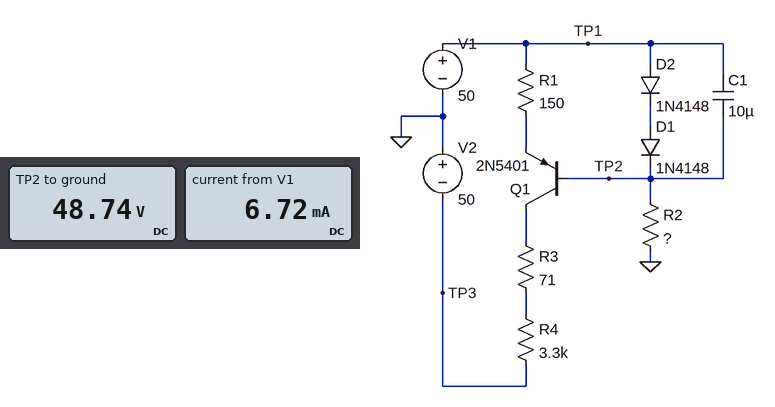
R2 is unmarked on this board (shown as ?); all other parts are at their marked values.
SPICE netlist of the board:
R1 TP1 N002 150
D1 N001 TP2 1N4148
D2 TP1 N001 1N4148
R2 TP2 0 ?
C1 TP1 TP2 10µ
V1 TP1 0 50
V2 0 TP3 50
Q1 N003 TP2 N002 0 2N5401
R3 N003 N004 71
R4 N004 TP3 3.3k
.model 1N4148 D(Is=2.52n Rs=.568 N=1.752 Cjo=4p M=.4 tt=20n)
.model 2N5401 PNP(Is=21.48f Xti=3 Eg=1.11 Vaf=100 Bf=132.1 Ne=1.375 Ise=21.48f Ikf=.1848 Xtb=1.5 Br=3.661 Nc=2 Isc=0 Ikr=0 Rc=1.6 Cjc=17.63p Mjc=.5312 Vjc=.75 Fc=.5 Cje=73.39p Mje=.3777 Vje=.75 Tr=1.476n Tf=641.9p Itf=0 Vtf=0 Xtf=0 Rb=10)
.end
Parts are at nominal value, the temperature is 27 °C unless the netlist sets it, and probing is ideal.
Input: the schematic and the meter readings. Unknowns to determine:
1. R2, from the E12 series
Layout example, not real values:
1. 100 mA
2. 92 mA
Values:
1. 18 kΩ
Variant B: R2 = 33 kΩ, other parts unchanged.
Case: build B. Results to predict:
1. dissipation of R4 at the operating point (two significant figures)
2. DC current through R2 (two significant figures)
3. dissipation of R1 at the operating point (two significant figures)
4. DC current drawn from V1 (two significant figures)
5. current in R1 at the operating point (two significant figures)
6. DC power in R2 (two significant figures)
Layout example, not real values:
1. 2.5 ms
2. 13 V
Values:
1. 44 mW
2. 1.5 mA
3. 2.0 mW
4. 5.1 mA
5. 3.7 mA
6. 72 mW
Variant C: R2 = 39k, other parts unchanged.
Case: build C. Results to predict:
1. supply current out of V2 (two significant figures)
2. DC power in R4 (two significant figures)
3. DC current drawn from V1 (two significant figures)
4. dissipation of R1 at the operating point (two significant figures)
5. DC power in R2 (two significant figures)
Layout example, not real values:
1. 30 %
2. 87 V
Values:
1. 3.6 mA
2. 42 mW
3. 4.8 mA
4. 1.9 mW
5. 61 mW
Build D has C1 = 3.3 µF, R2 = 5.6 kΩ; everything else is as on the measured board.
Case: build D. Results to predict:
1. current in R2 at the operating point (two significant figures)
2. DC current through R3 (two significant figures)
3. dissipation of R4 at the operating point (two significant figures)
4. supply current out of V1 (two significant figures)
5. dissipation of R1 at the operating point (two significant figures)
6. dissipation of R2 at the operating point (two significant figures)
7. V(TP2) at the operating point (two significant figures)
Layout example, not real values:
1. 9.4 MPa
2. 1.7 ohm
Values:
1. 8.7 mA
2. 4.7 mA
3. 74 mW
4. 13 mA
5. 3.4 mW
6. 420 mW
7. 49 V
